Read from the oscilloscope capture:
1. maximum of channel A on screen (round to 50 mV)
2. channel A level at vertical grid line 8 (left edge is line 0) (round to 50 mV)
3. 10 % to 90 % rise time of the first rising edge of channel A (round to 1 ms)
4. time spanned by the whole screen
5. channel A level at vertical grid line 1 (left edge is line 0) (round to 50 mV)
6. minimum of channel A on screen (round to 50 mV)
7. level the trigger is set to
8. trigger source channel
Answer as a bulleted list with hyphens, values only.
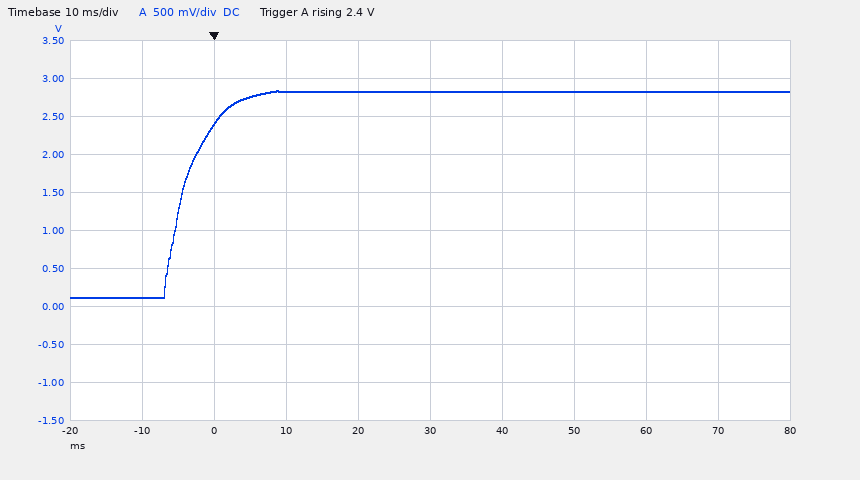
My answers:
- 2.85 V
- 2.85 V
- 8 ms
- 100 ms
- 100 mV
- 100 mV
- 2.4 V
- channel A
